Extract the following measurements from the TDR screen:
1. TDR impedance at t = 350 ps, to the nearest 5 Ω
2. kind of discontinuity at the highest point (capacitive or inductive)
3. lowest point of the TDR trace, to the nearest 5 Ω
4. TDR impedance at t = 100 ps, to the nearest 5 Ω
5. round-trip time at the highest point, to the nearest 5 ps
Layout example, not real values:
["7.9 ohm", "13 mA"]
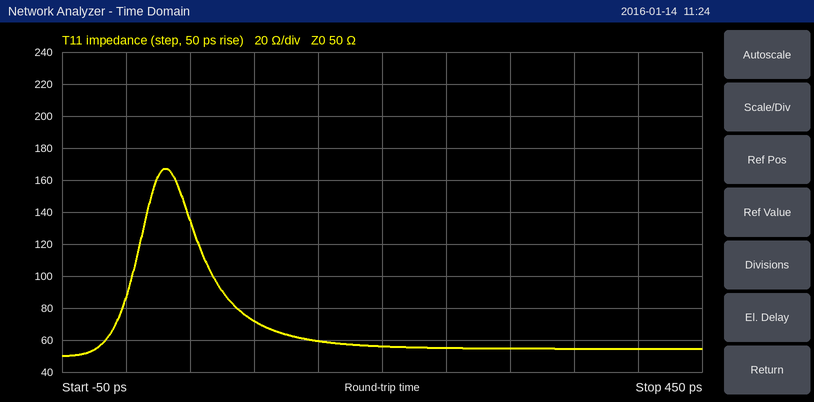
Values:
["55 Ω", "inductive", "50 Ω", "70 Ω", "30 ps"]
